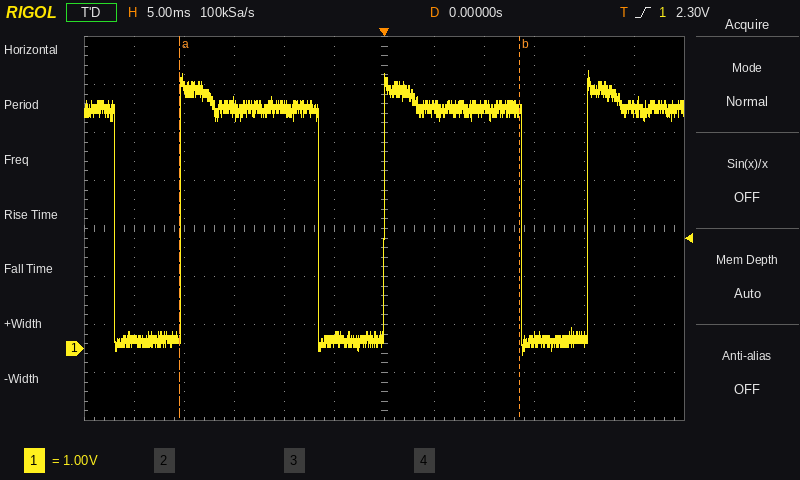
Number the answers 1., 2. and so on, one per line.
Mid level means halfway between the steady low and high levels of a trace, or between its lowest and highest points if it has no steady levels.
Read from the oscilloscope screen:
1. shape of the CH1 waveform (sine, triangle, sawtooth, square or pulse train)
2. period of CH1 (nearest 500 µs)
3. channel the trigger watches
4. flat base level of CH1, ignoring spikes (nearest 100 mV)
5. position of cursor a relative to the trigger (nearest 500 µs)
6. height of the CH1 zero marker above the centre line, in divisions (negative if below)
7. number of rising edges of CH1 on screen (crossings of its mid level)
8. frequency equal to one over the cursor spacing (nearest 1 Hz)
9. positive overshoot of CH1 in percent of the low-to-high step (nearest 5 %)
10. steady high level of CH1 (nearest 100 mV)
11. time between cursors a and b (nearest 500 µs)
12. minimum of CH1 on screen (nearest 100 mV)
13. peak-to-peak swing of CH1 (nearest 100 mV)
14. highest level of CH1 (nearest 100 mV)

1. pulse train
2. 20.5 ms
3. CH1
4. 200 mV
5. -20.5 ms
6. -2.5 div
7. 3
8. 29 Hz
9. 15 %
10. 5.0 V
11. 34.0 ms
12. -100 mV
13. 5.9 V
14. 5.8 V
